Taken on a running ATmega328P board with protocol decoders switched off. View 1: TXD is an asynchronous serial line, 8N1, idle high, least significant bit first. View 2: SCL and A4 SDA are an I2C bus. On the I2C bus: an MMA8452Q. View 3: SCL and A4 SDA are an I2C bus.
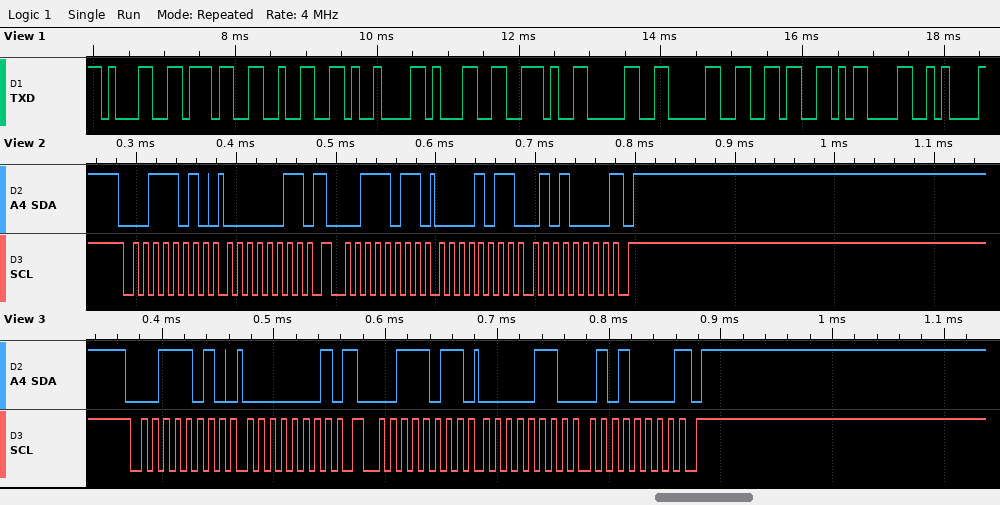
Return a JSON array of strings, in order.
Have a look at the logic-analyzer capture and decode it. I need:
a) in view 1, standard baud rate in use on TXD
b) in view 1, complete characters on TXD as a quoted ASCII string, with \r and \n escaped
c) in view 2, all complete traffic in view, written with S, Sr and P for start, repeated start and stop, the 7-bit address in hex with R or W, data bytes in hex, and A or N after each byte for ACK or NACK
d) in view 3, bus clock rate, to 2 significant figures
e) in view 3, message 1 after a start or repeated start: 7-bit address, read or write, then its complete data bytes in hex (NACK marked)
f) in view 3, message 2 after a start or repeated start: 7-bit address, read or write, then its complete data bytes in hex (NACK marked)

["9600 baud", "\"172\\t1.006\\r\\n\"", "S 1DW A 03 A Sr 1DR A 0B A 50 N P", "100 kHz", "0x1D write: 01", "0x1D read: 06 50 NACK"]
